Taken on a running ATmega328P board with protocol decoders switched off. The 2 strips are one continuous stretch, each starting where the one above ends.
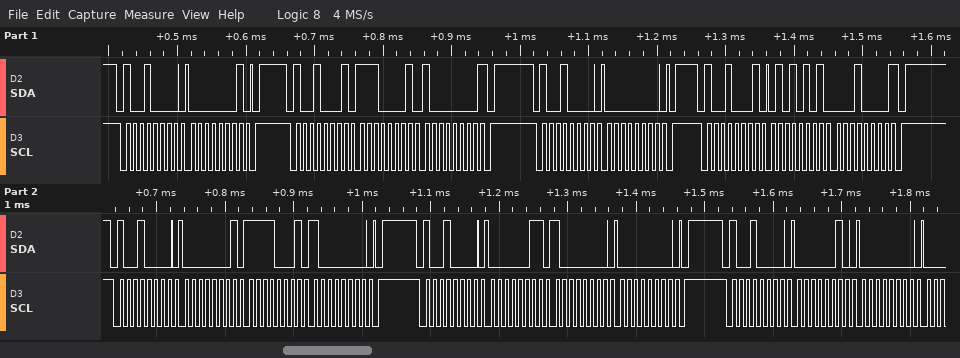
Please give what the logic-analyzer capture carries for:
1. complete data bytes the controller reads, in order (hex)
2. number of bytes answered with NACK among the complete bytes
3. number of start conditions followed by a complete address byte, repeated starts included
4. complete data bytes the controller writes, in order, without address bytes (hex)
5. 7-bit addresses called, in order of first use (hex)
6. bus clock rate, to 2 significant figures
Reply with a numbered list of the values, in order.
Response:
1. E1 80 55 10
2. 2
3. 7
4. 01 00 01 F1 80 03 80 00 02 00
5. 0x48
6. 100 kHz
